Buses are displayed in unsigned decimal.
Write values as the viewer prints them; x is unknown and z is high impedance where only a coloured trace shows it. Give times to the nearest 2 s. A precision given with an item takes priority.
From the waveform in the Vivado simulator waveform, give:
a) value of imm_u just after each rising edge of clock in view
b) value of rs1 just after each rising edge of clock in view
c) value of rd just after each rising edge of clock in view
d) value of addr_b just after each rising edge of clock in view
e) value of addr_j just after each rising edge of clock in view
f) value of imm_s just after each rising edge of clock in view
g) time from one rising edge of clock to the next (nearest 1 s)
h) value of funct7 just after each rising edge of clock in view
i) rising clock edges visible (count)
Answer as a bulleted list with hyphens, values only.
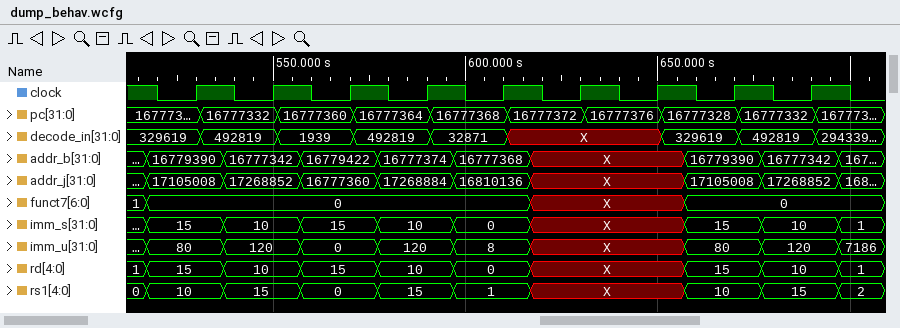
- 80, 120, 0, 120, 8, X, X, 80, 120
- 10, 15, 0, 15, 1, X, X, 10, 15
- 15, 10, 15, 10, 0, X, X, 15, 10
- 16779390, 16777342, 16779422, 16777374, 16777368, X, X, 16779390, 16777342
- 17105008, 17268852, 16777360, 17268884, 16810136, X, X, 17105008, 17268852
- 15, 10, 15, 10, 0, X, X, 15, 10
- 20 s
- 0, 0, 0, 0, 0, X, X, 0, 0
- 9
